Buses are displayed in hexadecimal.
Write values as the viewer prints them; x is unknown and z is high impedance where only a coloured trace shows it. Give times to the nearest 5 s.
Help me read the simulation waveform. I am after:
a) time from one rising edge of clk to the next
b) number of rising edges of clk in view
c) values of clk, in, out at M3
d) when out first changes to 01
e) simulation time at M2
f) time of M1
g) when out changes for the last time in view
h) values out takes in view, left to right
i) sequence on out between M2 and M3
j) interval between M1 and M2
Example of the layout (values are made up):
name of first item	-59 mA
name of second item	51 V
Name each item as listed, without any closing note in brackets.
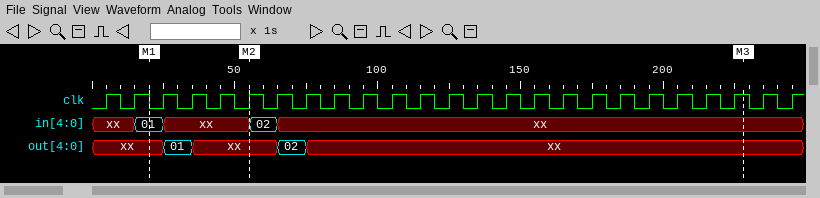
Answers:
time from one rising edge of clk to the next	10 s
number of rising edges of clk in view	25
values of clk, in, out at M3	clk=1, in=xx, out=xx
when out first changes to 01	25 s
simulation time at M2	55 s
time of M1	20 s
when out changes for the last time in view	75 s
values out takes in view, left to right	xx, 01, xx, 02, xx
sequence on out between M2 and M3	xx, 02, xx
interval between M1 and M2	35 s
